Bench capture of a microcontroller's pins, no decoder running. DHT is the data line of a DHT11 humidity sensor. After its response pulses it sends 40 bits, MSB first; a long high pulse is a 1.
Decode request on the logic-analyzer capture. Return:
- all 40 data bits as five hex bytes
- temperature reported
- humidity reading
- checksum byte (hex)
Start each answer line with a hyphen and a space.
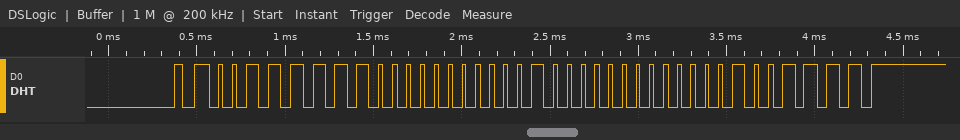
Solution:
- 3F 00 10 00 4F
- 16.0 °C
- 63 %
- 0x4F
